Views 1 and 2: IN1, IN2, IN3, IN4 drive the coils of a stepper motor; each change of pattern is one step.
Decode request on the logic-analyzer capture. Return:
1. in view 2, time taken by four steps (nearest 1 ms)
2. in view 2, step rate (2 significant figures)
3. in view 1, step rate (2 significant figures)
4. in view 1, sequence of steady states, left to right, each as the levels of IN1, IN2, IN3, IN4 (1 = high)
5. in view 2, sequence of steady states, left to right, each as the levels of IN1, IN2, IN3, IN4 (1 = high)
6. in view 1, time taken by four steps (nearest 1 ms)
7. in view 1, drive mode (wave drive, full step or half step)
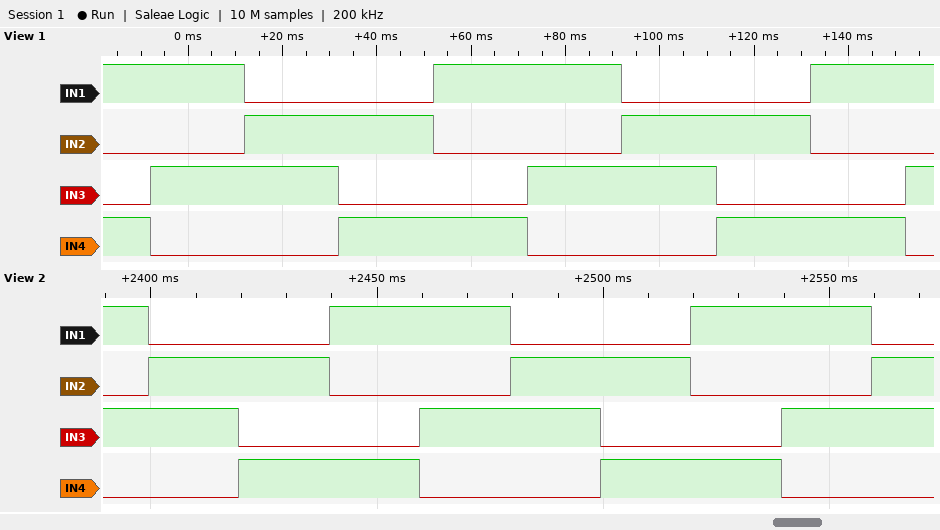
80 ms
50 steps/s
50 steps/s
1001 1010 0110 0101 1001 1010 0110 0101 1001 1010
1010 0110 0101 1001 1010 0110 0101 1001 1010 0110
80 ms
full step
